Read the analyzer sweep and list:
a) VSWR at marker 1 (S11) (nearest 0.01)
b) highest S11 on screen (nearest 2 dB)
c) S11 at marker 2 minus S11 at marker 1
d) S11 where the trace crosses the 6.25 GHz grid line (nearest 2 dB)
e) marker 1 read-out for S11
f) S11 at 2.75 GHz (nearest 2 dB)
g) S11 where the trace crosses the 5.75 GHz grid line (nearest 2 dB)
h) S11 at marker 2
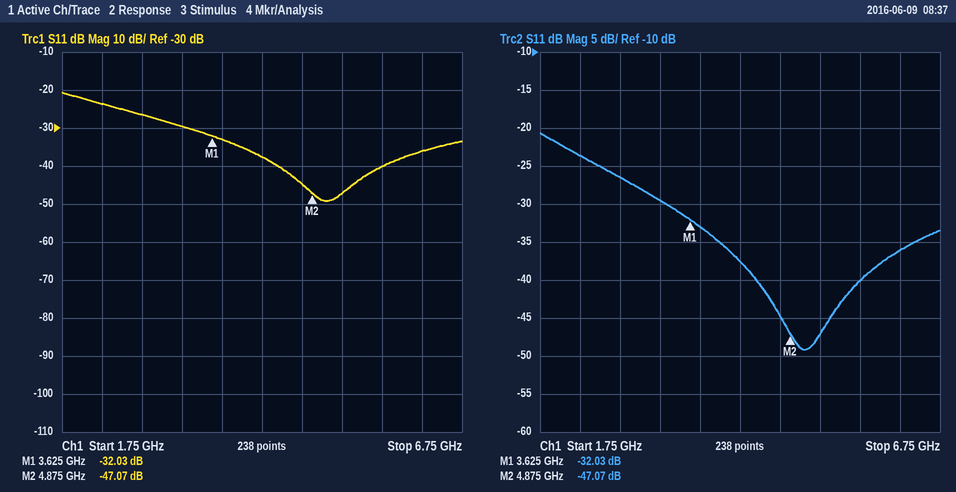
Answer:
1.05
-20 dB
-15.04 dB
-36 dB
-32.03 dB
-26 dB
-40 dB
-47.07 dB
